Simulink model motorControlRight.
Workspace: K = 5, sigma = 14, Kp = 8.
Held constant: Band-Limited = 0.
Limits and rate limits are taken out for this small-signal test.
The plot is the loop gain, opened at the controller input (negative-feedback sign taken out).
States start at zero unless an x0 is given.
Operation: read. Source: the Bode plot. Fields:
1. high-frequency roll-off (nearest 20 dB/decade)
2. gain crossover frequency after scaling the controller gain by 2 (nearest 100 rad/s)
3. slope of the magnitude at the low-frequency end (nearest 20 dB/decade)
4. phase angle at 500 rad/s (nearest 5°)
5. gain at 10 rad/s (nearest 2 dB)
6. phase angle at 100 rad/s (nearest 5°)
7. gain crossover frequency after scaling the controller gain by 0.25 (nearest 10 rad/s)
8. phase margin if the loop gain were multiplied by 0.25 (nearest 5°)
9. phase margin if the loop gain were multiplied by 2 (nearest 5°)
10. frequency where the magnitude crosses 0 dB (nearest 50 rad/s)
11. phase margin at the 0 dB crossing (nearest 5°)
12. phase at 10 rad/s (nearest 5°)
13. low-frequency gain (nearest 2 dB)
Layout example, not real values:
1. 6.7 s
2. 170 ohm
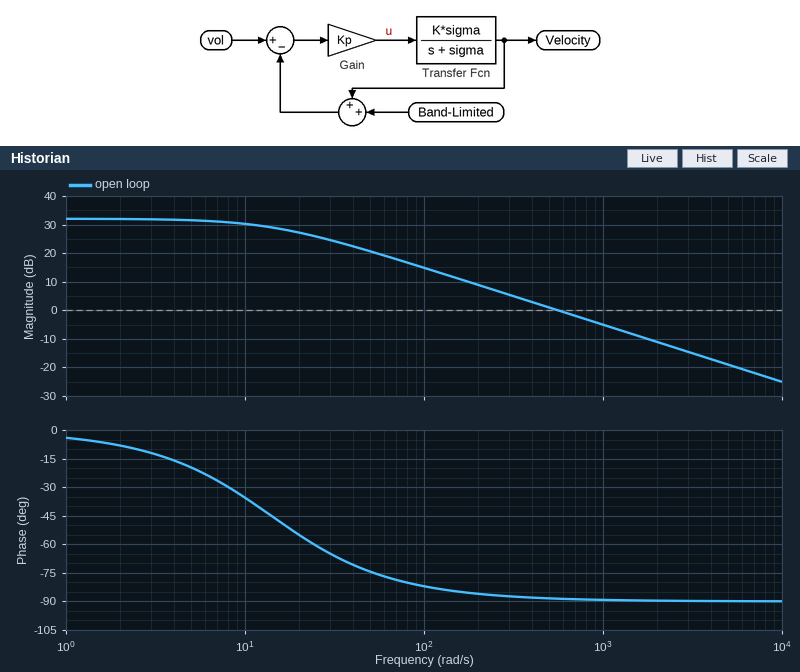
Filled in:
1. -20 dB/decade
2. 1100 rad/s
3. 0 dB/decade
4. -90°
5. 30 dB
6. -80°
7. 140 rad/s
8. 95°
9. 90°
10. 550 rad/s
11. 90°
12. -35°
13. 32 dB
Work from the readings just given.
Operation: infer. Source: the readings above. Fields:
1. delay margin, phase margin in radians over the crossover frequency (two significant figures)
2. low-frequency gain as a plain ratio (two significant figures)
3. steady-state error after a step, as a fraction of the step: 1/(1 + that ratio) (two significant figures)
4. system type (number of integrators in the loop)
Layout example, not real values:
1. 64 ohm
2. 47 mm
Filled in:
1. 0.0029 s
2. 40
3. 0.024
4. 0
